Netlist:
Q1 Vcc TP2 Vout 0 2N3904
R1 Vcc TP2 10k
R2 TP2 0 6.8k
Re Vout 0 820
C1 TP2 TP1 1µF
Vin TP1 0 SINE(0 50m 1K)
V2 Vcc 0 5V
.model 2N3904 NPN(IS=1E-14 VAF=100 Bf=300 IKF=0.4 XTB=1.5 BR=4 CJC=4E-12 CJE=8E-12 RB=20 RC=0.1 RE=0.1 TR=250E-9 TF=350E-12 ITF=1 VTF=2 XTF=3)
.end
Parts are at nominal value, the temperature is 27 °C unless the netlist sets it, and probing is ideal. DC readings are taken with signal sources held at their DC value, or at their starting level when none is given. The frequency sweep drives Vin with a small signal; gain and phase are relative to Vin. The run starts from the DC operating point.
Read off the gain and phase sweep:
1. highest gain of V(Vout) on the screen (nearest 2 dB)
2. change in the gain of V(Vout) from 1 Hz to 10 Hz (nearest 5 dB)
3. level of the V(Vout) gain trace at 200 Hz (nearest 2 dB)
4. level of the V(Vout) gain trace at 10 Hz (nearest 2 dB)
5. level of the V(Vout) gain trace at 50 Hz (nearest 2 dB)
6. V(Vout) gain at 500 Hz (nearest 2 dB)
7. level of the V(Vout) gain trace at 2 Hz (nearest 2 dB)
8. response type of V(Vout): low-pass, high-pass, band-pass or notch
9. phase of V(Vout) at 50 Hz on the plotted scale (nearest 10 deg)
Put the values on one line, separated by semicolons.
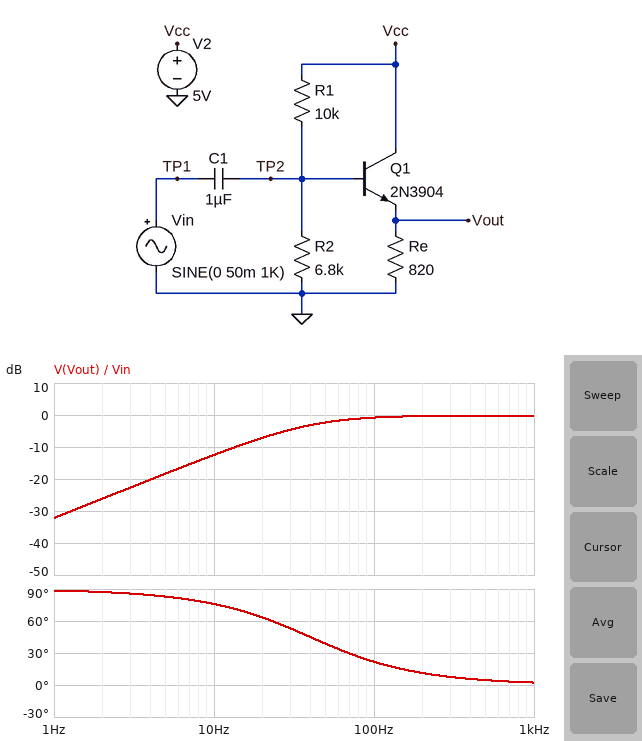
0 dB; 20 dB; 0 dB; -12 dB; -2 dB; 0 dB; -26 dB; high-pass; 40 deg
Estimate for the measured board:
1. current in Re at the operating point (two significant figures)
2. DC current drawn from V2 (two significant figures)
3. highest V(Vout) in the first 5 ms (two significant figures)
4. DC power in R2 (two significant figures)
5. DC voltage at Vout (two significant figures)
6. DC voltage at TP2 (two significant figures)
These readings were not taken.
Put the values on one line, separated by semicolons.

1.6 mA; 1.9 mA; 1.4 V; 590 µW; 1.3 V; 2.0 V
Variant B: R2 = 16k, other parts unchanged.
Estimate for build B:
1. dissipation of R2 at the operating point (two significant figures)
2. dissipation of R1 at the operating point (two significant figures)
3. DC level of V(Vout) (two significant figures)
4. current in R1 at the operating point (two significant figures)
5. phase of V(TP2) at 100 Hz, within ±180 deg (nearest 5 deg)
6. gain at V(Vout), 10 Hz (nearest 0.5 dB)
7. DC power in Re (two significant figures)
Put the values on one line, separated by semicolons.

570 µW; 390 µW; 2.3 V; 200 µA; 15 deg; -9.0 dB; 6.7 mW
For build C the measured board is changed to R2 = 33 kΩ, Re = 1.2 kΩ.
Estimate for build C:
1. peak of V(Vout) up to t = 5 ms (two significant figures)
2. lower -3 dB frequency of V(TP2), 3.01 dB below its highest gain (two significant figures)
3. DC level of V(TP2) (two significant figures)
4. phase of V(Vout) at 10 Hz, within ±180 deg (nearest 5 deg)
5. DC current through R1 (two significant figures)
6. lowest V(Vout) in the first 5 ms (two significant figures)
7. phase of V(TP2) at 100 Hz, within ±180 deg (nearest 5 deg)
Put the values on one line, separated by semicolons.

3.1 V; 21 Hz; 3.8 V; 65 deg; 120 µA; 3.0 V; 10 deg
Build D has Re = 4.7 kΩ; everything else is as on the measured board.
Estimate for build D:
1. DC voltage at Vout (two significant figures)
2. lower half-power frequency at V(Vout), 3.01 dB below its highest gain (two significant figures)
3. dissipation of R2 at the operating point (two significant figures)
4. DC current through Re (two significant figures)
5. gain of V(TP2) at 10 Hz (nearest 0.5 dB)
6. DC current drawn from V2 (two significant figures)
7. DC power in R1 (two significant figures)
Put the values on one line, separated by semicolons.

1.4 V; 39 Hz; 600 µW; 300 µA; -12.0 dB; 590 µA; 890 µW
